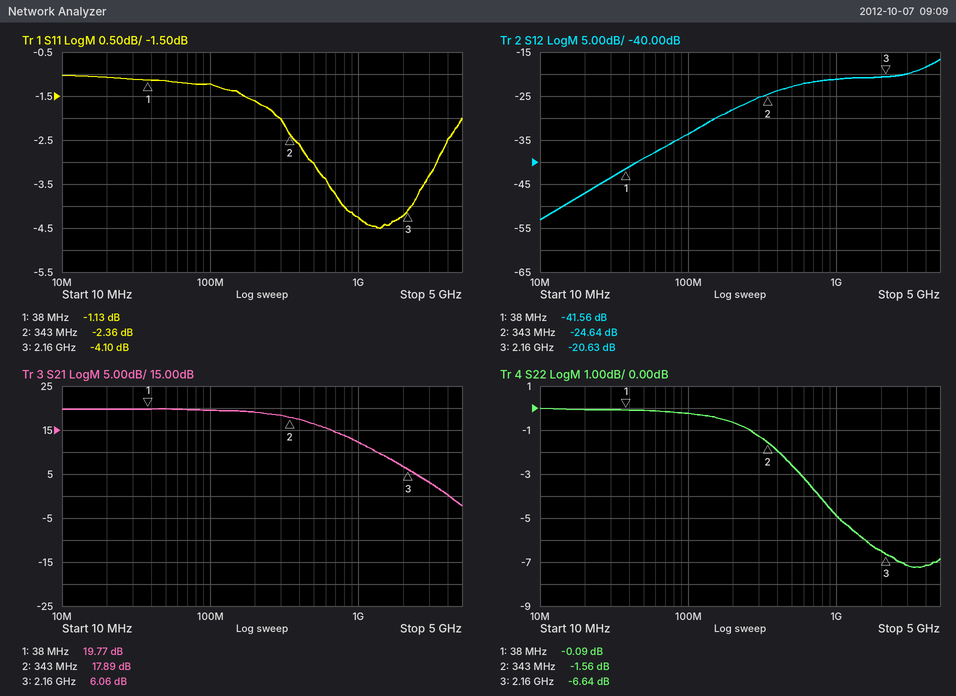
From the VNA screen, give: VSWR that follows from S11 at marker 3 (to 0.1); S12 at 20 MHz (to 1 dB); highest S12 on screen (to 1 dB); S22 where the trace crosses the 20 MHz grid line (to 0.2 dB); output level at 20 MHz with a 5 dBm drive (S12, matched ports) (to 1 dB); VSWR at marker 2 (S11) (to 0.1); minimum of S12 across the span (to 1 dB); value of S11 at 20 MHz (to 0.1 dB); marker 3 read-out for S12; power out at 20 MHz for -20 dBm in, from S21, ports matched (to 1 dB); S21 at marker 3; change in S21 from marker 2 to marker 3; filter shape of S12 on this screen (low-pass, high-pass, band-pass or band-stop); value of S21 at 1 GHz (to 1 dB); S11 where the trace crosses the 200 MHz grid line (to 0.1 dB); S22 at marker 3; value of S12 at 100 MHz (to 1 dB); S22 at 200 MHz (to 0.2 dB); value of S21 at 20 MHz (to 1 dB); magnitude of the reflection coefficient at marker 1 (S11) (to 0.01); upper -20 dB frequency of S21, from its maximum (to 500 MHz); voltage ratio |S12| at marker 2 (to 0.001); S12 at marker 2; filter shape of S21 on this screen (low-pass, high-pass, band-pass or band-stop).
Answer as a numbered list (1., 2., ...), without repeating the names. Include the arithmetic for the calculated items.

1. (1 + 0.6237)/(1 − 0.6237) ≈ 4.3
2. -47 dB
3. -17 dB
4. 0.0 dB
5. 5 dBm + (-47 dB) = -42 dBm
6. (1 + 0.7621)/(1 − 0.7621) ≈ 7.4
7. -53 dB
8. -1.1 dB
9. -20.63 dB
10. -20 dBm + (20 dB) = 0 dBm
11. 6.06 dB
12. 6.06 − (17.89) = -11.83 dB
13. high-pass
14. 12 dB
15. -1.6 dB
16. -6.64 dB
17. -34 dB
18. -0.6 dB
19. 20 dB
20. 10^(-1.13/20) ≈ 0.88
21. 4.0 GHz
22. 10^(-24.64/20) ≈ 0.059
23. -24.64 dB
24. low-pass
